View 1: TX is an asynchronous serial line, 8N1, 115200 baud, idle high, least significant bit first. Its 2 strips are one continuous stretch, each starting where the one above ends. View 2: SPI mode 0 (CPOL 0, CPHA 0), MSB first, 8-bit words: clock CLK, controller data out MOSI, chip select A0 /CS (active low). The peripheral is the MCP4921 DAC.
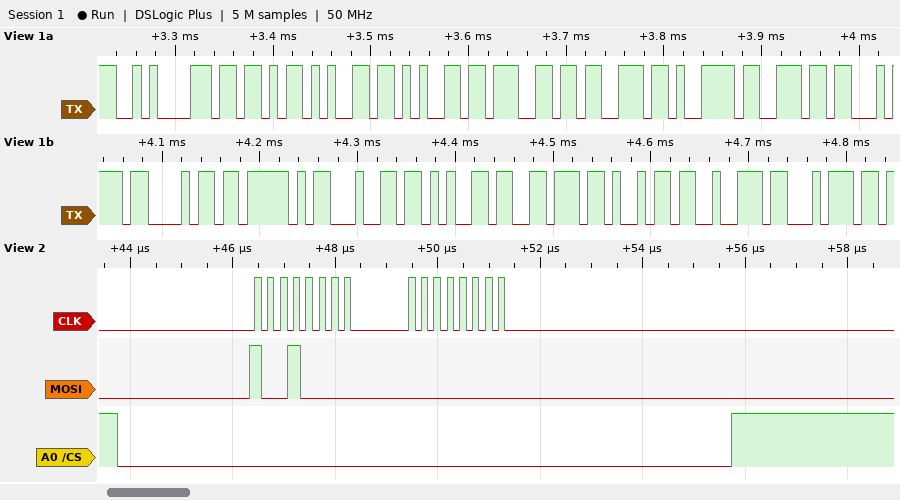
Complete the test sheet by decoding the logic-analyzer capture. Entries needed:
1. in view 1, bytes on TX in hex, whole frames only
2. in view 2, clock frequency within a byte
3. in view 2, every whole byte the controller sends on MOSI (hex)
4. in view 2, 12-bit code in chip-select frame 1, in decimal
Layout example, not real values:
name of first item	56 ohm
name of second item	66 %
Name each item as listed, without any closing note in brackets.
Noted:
in view 1, bytes on TX in hex, whole frames only	0A 5B 65 65 67 73 79 6E 74 68 5F 64 65 76 69 72 74
in view 2, clock frequency within a byte	4 MHz
in view 2, every whole byte the controller sends on MOSI	90 00
in view 2, 12-bit code in chip-select frame 1, in decimal	0
